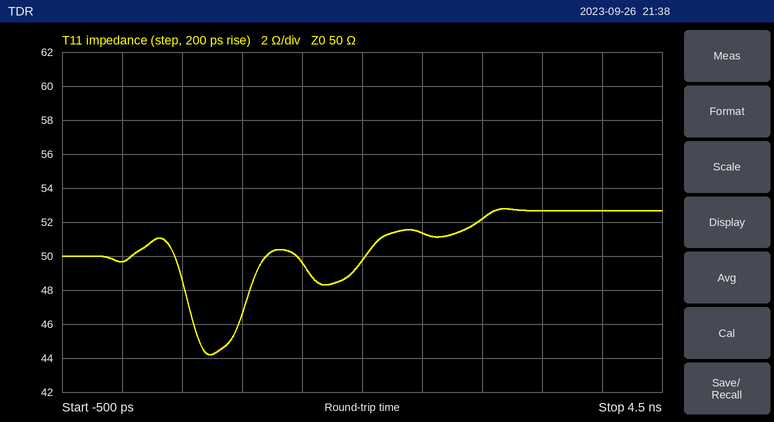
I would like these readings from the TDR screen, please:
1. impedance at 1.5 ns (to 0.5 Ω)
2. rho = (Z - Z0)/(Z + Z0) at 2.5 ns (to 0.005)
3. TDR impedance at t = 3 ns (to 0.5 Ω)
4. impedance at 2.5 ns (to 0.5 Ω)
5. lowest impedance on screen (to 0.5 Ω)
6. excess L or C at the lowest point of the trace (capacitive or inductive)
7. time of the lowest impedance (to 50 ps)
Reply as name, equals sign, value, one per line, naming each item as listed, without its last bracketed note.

impedance at 1.5 ns = 49.5 Ω
rho = (Z - Z0)/(Z + Z0) at 2.5 ns = +0.015
TDR impedance at t = 3 ns = 52.0 Ω
impedance at 2.5 ns = 51.5 Ω
lowest impedance on screen = 44.0 Ω
excess L or C at the lowest point of the trace = capacitive
time of the lowest impedance = 750 ps
